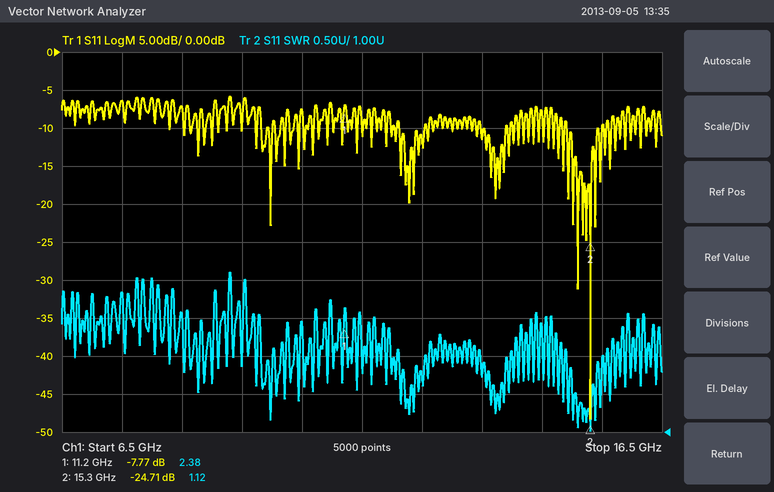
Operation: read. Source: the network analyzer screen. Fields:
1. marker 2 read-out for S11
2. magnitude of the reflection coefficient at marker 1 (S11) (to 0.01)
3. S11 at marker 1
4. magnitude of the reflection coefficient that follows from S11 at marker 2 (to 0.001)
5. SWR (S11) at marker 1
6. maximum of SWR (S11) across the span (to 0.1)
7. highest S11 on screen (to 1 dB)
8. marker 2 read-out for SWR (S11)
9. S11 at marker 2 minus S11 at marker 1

-24.71 dB
0.41
-7.77 dB
0.058
2.38
3.1
-6 dB
1.12
-16.94 dB
